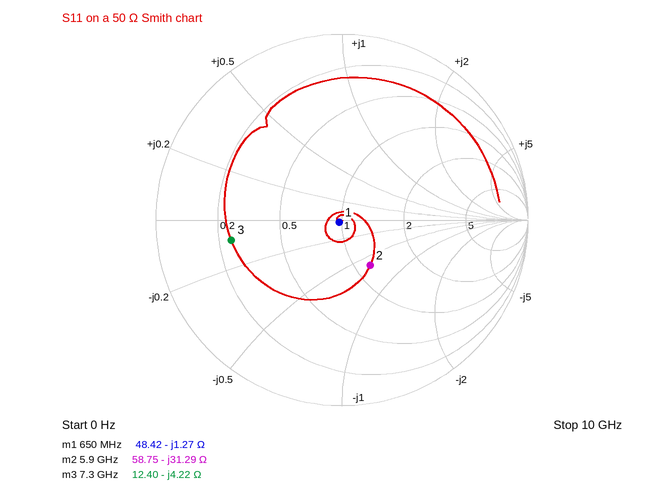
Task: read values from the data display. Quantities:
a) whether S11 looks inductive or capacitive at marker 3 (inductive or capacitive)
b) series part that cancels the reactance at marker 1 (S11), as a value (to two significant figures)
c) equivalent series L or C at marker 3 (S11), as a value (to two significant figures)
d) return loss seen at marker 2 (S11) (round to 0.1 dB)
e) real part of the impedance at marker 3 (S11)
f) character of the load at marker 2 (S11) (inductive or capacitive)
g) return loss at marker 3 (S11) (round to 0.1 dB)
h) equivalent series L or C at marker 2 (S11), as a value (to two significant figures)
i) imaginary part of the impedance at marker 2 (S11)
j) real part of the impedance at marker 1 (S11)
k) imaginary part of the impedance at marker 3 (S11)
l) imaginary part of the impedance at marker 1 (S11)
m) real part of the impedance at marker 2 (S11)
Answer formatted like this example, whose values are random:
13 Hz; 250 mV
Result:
capacitive; 310 pH; 5.2 pF; 10.8 dB; 12.40 Ω; capacitive; 4.4 dB; 860 fF; -31.29 Ω; 48.42 Ω; -4.22 Ω; -1.27 Ω; 58.75 Ω
